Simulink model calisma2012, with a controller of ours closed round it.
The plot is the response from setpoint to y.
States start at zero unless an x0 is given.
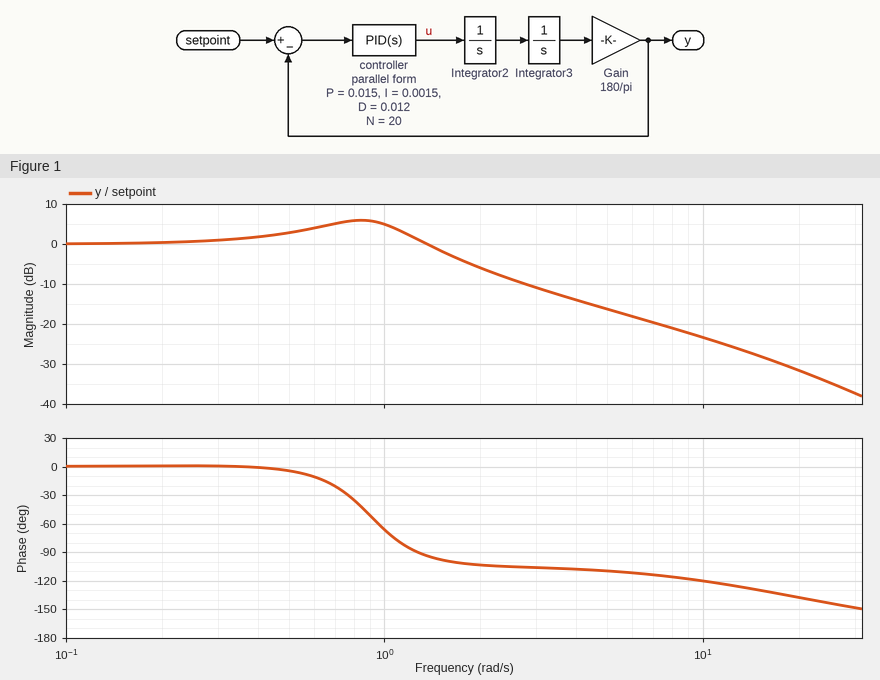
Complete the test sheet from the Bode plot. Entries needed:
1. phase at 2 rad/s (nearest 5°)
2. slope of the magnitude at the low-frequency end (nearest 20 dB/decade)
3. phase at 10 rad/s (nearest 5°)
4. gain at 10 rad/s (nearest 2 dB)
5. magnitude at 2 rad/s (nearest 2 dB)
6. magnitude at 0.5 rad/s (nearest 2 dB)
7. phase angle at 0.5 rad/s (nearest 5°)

-105°
0 dB/decade
-120°
-24 dB
-6 dB
2 dB
-5°
